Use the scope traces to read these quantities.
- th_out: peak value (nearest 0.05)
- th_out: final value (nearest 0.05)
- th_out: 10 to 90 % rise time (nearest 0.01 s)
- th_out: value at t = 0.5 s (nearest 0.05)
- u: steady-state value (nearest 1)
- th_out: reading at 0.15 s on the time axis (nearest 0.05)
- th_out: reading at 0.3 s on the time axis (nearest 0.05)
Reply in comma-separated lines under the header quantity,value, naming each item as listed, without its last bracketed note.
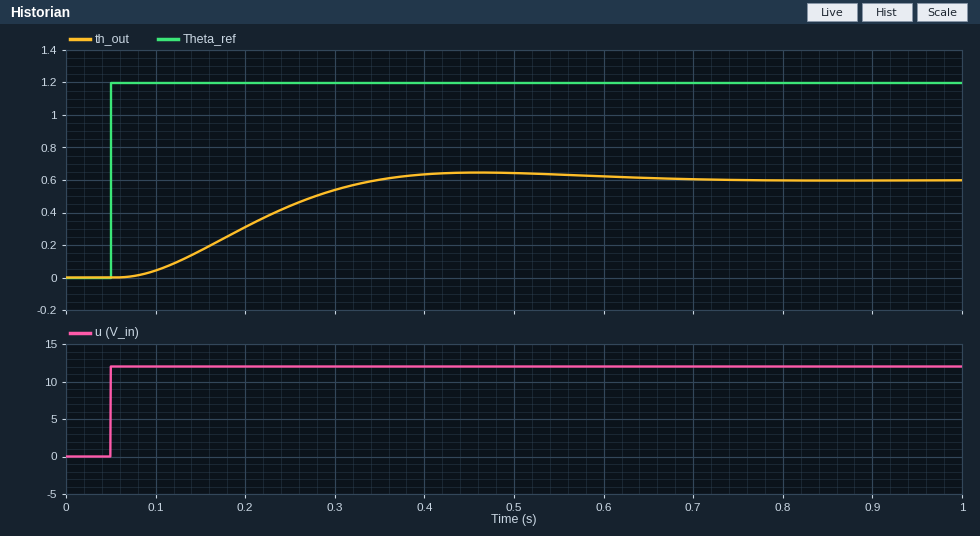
quantity,value
th_out: peak value,0.65
th_out: final value,0.60
th_out: 10 to 90 % rise time,0.19 s
th_out: value at t = 0.5 s,0.65
u: steady-state value,12
th_out: reading at 0.15 s on the time axis,0.15
th_out: reading at 0.3 s on the time axis,0.55
